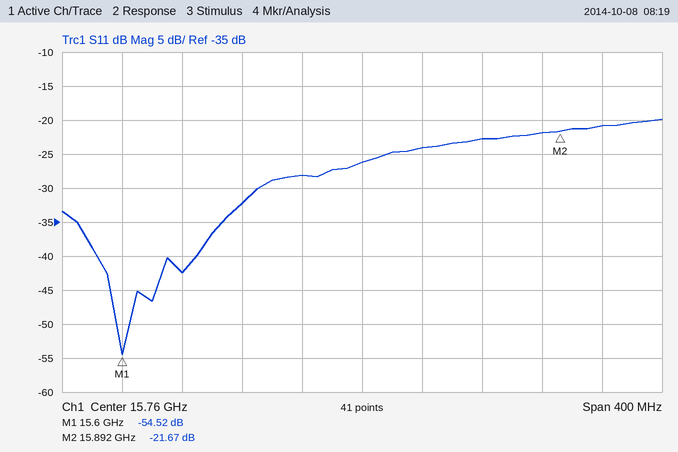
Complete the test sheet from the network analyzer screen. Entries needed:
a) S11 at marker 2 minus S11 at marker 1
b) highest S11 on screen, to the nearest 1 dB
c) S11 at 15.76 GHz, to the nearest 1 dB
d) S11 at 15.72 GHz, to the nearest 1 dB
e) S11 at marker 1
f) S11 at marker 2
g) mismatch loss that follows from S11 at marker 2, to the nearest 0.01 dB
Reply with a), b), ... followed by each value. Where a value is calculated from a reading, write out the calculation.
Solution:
a) -21.67 − (-54.52) = 32.85 dB
b) -20 dB
c) -26 dB
d) -28 dB
e) -54.52 dB
f) -21.67 dB
g) −10 log10(1 − 10^(-21.67/10)) ≈ 0.03 dB
